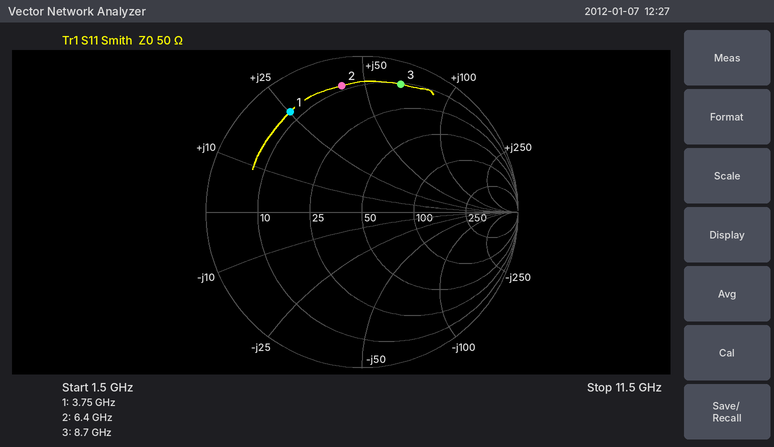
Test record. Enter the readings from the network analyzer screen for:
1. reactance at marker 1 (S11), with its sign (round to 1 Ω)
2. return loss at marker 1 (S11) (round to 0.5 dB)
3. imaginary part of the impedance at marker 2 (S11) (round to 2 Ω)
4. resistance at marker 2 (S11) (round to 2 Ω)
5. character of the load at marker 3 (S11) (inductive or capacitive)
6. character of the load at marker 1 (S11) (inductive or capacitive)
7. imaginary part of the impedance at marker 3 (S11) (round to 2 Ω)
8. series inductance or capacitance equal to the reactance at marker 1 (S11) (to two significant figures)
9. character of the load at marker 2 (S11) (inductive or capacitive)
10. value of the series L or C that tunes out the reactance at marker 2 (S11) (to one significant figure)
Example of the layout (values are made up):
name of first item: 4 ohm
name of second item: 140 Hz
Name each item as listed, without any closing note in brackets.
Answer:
reactance at marker 1 (S11), with its sign: +25 Ω
return loss at marker 1 (S11): 2.0 dB
imaginary part of the impedance at marker 2 (S11): +42 Ω
resistance at marker 2 (S11): 8 Ω
character of the load at marker 3 (S11): inductive
character of the load at marker 1 (S11): inductive
imaginary part of the impedance at marker 3 (S11): +66 Ω
series inductance or capacitance equal to the reactance at marker 1 (S11): 1.1 nH
character of the load at marker 2 (S11): inductive
value of the series L or C that tunes out the reactance at marker 2 (S11): 600 fF
